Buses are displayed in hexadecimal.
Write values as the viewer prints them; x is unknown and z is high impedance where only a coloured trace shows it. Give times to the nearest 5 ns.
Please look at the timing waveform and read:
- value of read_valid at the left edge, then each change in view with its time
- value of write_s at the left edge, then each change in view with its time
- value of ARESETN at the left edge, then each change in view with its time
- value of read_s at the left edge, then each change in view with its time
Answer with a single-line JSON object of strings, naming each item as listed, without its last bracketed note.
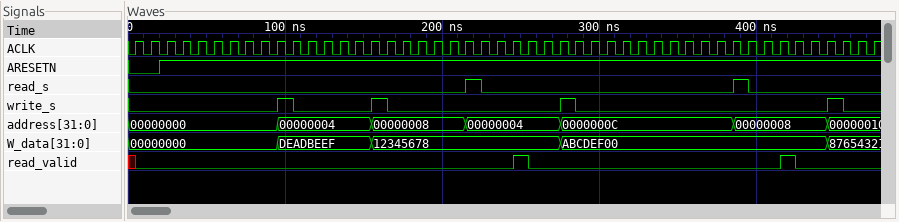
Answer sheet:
{"value of read_valid at the left edge, then each change in view with its time": "x, 0 at 5 ns, 1 at 245 ns, 0 at 255 ns, 1 at 415 ns, 0 at 425 ns", "value of write_s at the left edge, then each change in view with its time": "0, 1 at 95 ns, 0 at 105 ns, 1 at 155 ns, 0 at 165 ns, 1 at 275 ns, 0 at 285 ns, 1 at 445 ns, 0 at 455 ns", "value of ARESETN at the left edge, then each change in view with its time": "0, 1 at 20 ns", "value of read_s at the left edge, then each change in view with its time": "0, 1 at 215 ns, 0 at 225 ns, 1 at 385 ns, 0 at 395 ns"}
